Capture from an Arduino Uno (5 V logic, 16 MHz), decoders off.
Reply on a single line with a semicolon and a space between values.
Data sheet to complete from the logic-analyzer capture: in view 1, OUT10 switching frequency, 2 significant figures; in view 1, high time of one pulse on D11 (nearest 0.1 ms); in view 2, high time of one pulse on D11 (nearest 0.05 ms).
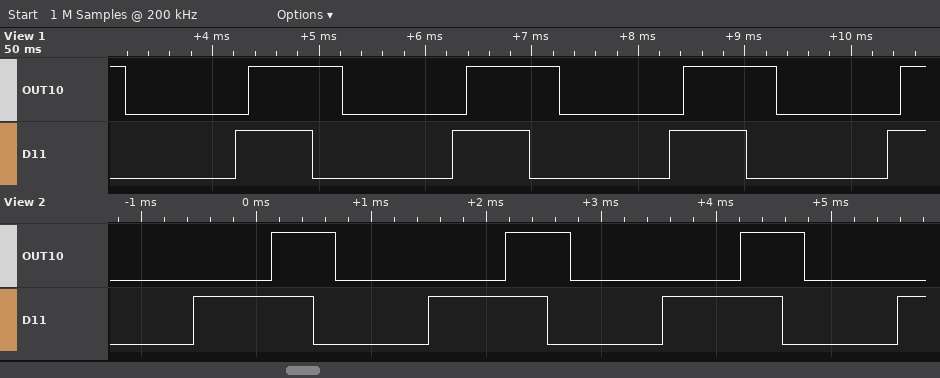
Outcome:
490 Hz; 0.7 ms; 1.05 ms
